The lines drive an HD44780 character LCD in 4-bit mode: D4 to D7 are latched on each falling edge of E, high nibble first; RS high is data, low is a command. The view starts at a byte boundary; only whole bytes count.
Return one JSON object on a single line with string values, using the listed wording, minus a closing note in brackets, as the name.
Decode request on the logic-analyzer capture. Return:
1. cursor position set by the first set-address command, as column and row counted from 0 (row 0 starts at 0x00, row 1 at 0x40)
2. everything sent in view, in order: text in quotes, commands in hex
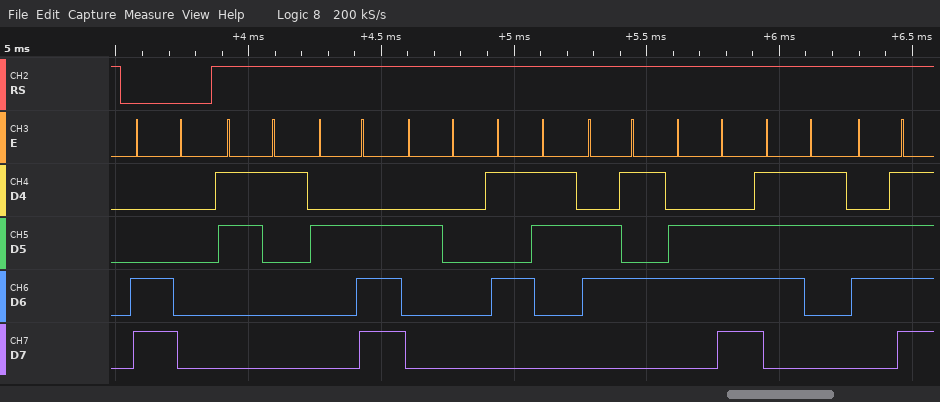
{"cursor position set by the first set-address command, as column and row counted from 0": "column 0, row 1", "everything sent in view, in order: text in quotes, commands in hex": "0xC0 \"1. Senso\""}
